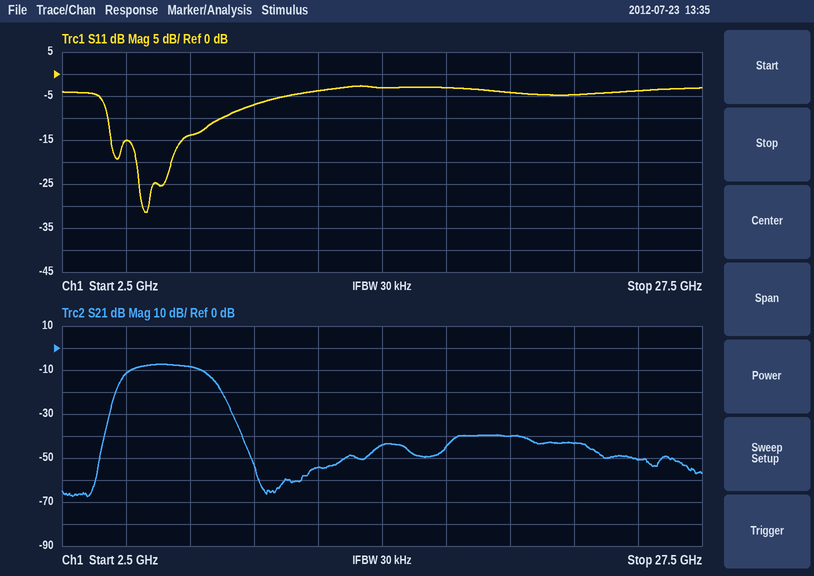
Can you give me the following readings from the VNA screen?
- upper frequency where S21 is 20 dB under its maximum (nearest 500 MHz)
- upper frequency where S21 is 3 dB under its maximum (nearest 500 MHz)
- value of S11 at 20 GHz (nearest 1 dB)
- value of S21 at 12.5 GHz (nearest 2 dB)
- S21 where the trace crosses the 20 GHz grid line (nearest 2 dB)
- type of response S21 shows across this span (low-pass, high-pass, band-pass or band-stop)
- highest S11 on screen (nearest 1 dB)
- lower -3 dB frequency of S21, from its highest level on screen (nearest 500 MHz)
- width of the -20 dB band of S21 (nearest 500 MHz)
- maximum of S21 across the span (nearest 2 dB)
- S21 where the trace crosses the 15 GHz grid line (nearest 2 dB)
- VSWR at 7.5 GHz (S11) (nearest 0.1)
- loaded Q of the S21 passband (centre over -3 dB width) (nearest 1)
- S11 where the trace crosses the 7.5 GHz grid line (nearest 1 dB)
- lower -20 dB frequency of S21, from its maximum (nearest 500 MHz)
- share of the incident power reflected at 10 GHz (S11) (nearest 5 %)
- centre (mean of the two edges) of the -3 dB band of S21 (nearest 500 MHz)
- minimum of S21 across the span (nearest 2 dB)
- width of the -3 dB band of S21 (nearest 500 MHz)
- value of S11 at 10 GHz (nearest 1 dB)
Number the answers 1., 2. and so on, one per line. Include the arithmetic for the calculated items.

1. 9.0 GHz
2. 8.0 GHz
3. -4 dB
4. -54 dB
5. -40 dB
6. band-pass
7. -3 dB
8. 5.0 GHz
9. 9.0 GHz − 4.5 GHz = 4.5 GHz
10. -8 dB
11. -44 dB
12. |Γ| = 10^(-14/20) = 0.1995; VSWR = (1 + 0.1995)/(1 − 0.1995) ≈ 1.5
13. 6.5 GHz / 3 GHz ≈ 2
14. -14 dB
15. 4.5 GHz
16. 10^(-7/10) ≈ 20 %
17. 6.5 GHz
18. -68 dB
19. 8.0 GHz − 5.0 GHz = 3.0 GHz
20. -7 dB
